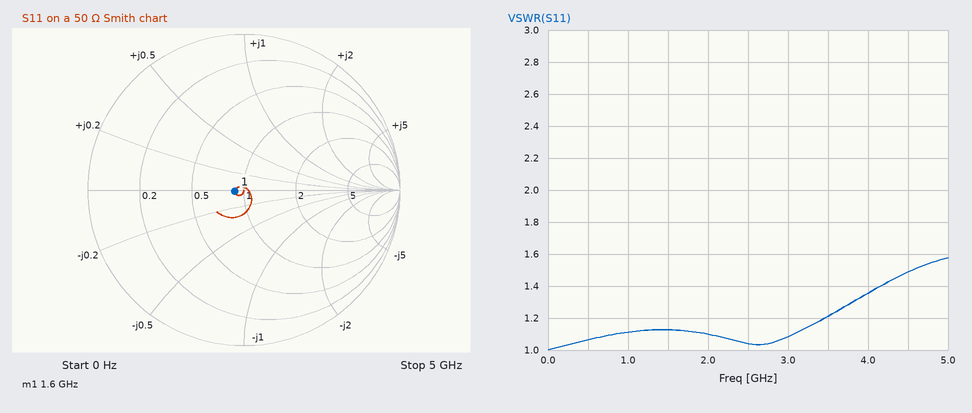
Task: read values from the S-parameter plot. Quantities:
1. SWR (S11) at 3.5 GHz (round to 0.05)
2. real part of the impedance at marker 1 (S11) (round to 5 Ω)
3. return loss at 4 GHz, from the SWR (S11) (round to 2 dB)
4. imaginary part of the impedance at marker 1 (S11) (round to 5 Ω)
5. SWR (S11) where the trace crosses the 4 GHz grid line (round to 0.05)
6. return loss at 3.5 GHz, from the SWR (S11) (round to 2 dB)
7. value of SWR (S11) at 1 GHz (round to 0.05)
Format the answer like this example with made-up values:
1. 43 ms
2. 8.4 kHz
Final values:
1. 1.20
2. 45 Ω
3. 16 dB
4. 0 Ω
5. 1.35
6. 20 dB
7. 1.10
